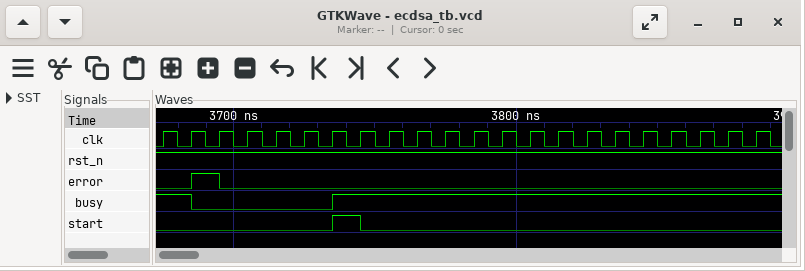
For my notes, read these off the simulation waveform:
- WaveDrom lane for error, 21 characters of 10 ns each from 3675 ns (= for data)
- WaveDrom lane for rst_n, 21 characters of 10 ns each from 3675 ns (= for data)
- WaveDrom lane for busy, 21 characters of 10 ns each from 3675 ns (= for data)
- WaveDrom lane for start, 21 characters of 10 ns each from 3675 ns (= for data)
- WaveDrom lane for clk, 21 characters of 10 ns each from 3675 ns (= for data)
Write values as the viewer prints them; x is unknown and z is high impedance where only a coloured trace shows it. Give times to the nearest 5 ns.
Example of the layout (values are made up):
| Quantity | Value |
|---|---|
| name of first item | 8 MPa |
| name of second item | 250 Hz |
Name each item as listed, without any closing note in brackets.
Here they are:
| Quantity | Value |
|---|---|
| WaveDrom lane for error, 21 characters of 10 ns each from 3675 ns | {name: 'error', wave: '010..................'} |
| WaveDrom lane for rst_n, 21 characters of 10 ns each from 3675 ns | {name: 'rst_n', wave: '1....................'} |
| WaveDrom lane for busy, 21 characters of 10 ns each from 3675 ns | {name: 'busy', wave: '10....1..............'} |
| WaveDrom lane for start, 21 characters of 10 ns each from 3675 ns | {name: 'start', wave: '0.....10.............'} |
| WaveDrom lane for clk, 21 characters of 10 ns each from 3675 ns | {name: 'clk', wave: 'p....................'} |
